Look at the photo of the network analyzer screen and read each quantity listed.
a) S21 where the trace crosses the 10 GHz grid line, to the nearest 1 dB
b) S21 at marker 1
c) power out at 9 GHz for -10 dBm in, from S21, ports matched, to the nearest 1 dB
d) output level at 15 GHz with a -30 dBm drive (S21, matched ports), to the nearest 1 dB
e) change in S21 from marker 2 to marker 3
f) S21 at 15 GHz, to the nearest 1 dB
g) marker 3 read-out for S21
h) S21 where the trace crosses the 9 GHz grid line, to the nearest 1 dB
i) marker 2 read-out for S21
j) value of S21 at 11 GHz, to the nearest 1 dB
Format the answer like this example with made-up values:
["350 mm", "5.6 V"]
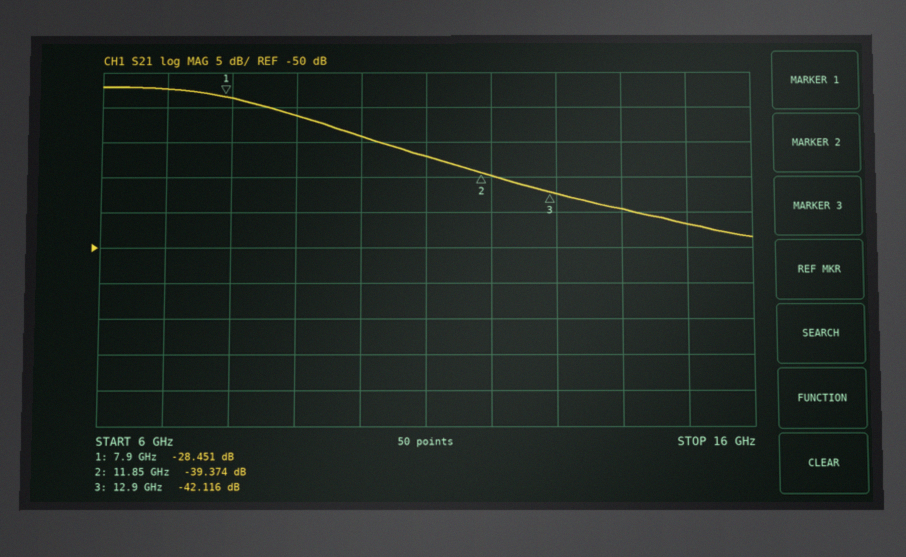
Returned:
["-34 dB", "-28.451 dB", "-41 dBm", "-77 dBm", "-2.742 dB", "-47 dB", "-42.116 dB", "-31 dB", "-39.374 dB", "-37 dB"]
